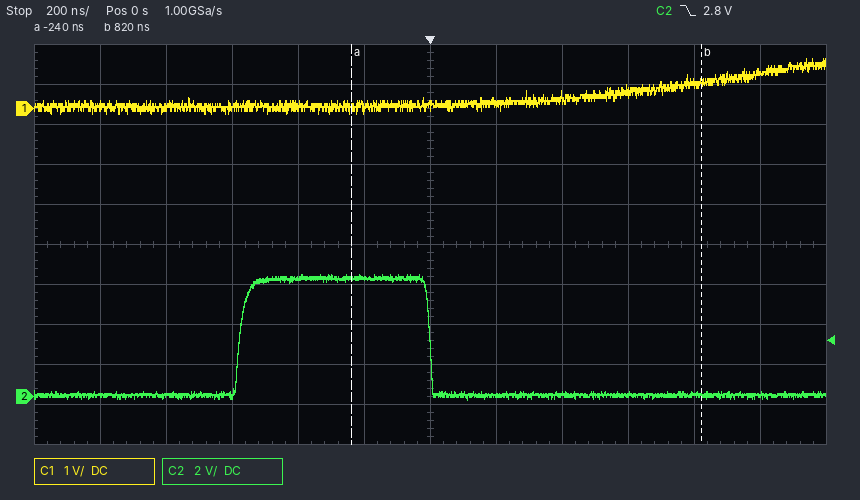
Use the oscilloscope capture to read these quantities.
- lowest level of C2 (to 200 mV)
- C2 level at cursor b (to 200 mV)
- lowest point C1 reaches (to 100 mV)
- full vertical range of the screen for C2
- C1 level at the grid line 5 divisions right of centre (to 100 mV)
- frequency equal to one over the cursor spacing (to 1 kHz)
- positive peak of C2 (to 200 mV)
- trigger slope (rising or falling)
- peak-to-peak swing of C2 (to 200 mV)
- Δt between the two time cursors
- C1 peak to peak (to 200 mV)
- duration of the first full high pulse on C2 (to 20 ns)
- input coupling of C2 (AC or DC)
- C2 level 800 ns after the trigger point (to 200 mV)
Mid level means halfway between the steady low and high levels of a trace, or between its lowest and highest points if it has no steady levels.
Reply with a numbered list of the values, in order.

1. -200 mV
2. 0.0 V
3. -100 mV
4. 20 V
5. 900 mV
6. 943 kHz
7. 6.0 V
8. falling
9. 6.2 V
10. 1.06 µs
11. 1.4 V
12. 580 ns
13. DC
14. 200 mV
